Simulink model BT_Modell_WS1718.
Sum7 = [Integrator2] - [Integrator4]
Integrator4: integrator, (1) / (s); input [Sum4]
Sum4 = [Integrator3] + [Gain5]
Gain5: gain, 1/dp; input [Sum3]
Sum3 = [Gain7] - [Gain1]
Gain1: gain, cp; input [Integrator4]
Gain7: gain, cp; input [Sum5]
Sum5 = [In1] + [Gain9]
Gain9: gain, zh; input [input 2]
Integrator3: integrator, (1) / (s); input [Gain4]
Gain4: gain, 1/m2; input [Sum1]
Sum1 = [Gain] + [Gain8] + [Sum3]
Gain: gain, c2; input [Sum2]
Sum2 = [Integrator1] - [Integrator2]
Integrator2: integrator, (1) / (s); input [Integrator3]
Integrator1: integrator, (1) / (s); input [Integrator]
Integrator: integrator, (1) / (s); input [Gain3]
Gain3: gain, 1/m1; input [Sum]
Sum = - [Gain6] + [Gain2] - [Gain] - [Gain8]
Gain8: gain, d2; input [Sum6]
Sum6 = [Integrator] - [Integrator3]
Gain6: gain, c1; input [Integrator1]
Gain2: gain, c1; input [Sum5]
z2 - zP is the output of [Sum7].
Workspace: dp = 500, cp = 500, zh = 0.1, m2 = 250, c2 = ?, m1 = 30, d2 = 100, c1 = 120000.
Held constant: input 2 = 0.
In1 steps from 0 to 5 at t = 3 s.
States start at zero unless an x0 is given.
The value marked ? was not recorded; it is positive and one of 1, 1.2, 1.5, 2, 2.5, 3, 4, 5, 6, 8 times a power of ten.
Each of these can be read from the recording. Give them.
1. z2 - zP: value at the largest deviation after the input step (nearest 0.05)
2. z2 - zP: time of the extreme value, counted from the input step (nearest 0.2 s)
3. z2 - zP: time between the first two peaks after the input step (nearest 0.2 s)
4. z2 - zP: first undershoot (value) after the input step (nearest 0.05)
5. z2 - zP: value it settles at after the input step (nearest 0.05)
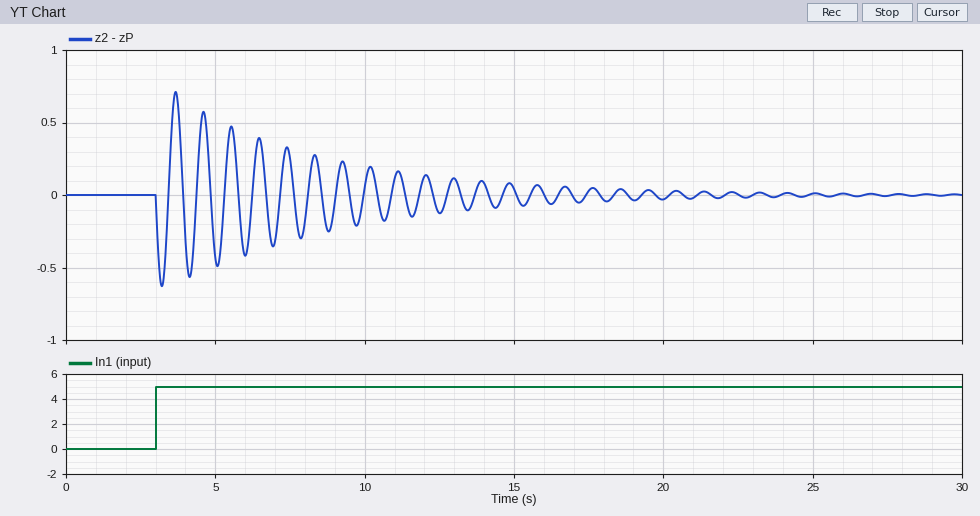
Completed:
0.70
0.6 s
1.0 s
-0.55
0.00
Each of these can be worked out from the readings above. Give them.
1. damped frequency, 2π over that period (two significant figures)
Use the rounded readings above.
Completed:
6.3 rad/s
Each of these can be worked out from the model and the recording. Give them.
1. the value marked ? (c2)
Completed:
12000
